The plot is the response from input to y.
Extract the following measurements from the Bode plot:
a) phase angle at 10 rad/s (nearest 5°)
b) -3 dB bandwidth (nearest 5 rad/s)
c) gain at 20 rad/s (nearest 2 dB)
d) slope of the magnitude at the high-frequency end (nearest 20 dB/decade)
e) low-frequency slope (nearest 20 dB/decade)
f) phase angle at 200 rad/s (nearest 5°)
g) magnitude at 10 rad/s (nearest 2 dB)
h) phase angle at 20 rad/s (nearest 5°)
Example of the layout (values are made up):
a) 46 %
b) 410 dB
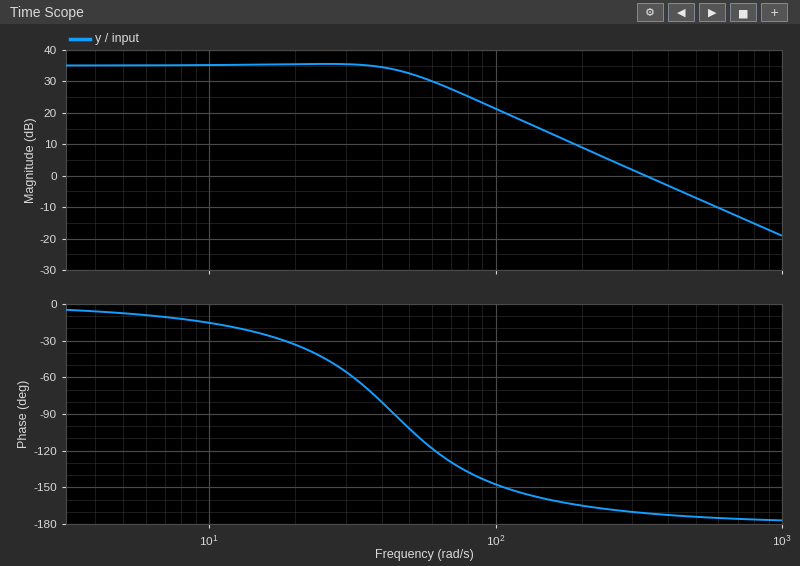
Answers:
a) -15°
b) 50 rad/s
c) 36 dB
d) -40 dB/decade
e) 0 dB/decade
f) -165°
g) 36 dB
h) -35°
